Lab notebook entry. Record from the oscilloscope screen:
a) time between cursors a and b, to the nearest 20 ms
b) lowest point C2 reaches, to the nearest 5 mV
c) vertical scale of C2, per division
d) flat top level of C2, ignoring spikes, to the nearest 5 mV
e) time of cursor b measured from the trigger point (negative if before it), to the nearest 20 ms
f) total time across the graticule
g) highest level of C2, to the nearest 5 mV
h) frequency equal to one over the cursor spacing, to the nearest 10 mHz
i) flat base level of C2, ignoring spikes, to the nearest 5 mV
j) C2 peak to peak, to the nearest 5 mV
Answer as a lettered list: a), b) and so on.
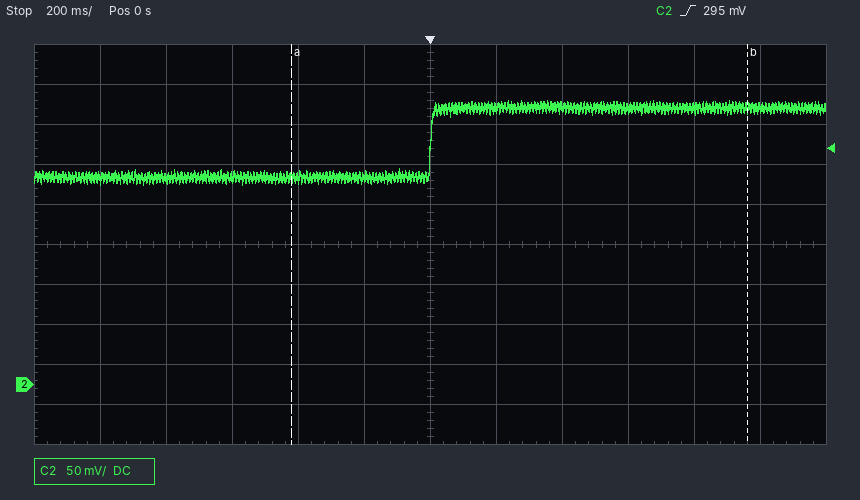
a) 1.38 s
b) 250 mV
c) 50 mV
d) 345 mV
e) +960 ms
f) 2.4 s
g) 355 mV
h) 720 mHz
i) 260 mV
j) 105 mV
